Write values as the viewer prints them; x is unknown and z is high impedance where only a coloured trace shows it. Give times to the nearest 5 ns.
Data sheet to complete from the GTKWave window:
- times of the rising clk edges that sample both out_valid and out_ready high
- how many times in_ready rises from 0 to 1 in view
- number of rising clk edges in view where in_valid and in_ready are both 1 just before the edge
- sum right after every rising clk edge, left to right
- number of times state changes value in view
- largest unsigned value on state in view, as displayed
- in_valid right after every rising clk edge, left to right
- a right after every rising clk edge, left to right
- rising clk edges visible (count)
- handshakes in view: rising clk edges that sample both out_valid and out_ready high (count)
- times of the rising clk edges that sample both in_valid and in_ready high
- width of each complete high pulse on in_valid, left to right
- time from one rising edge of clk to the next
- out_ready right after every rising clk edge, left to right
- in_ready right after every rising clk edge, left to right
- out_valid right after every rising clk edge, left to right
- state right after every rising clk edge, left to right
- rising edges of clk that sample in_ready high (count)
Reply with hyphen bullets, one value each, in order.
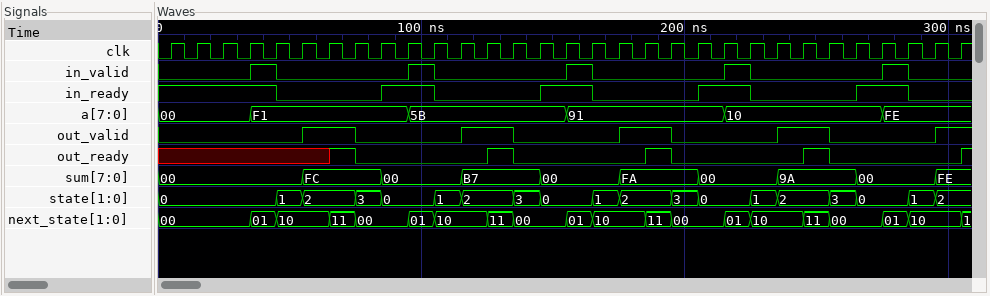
- 75 ns, 135 ns, 195 ns, 255 ns
- 4
- 5
- 00, 00, 00, 00, 00, FC, FC, FC, 00, 00, 00, B7, B7, B7, 00, 00, 00, FA, FA, FA, 00, 00, 00, 9A, 9A, 9A, 00, 00, 00, FE, FE
- 18
- 3
- 0 0 0 1 0 0 0 0 0 1 0 0 0 0 0 1 0 0 0 0 0 1 0 0 0 0 0 1 0 0 0
- 00, 00, 00, F1, F1, F1, F1, F1, F1, 5B, 5B, 5B, 5B, 5B, 5B, 91, 91, 91, 91, 91, 91, 10, 10, 10, 10, 10, 10, FE, FE, FE, FE
- 31
- 4
- 45 ns, 105 ns, 165 ns, 225 ns, 285 ns
- 10 ns, 10 ns, 10 ns, 10 ns, 10 ns
- 10 ns
- x x x x x x 1 0 0 0 0 0 1 0 0 0 0 0 1 0 0 0 0 0 1 0 0 0 0 0 1
- 1 1 1 1 0 0 0 0 1 1 0 0 0 0 1 1 0 0 0 0 1 1 0 0 0 0 1 1 0 0 0
- 0 0 0 0 0 1 1 0 0 0 0 1 1 0 0 0 0 1 1 0 0 0 0 1 1 0 0 0 0 1 1
- 0, 0, 0, 0, 1, 2, 2, 3, 0, 0, 1, 2, 2, 3, 0, 0, 1, 2, 2, 3, 0, 0, 1, 2, 2, 3, 0, 0, 1, 2, 2
- 13
